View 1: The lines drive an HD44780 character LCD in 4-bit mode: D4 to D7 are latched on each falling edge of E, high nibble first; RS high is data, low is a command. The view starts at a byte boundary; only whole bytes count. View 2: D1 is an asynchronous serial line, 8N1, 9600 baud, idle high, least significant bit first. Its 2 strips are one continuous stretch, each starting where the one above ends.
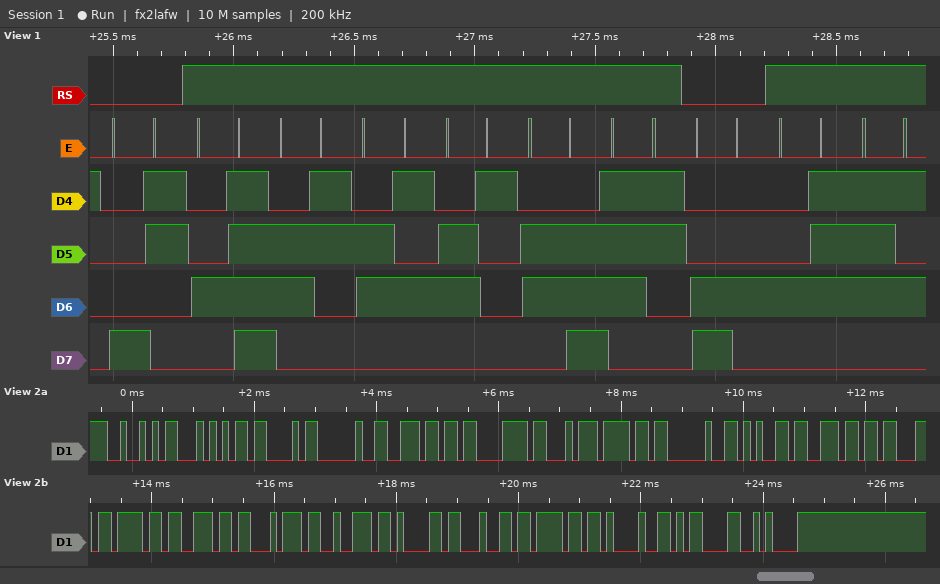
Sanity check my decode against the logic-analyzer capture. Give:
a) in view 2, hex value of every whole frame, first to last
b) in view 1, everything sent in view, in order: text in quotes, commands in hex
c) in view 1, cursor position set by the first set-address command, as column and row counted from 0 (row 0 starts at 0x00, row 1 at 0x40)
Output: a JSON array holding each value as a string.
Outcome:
["52 54 43 20 6E C3 A3 6F 20 65 6E 63 6F 6E 74 72 61 64 6F 21 0D 0A", "0x83 \"Oceans\" 0xC4 \"Gu\"", "column 3, row 0"]
